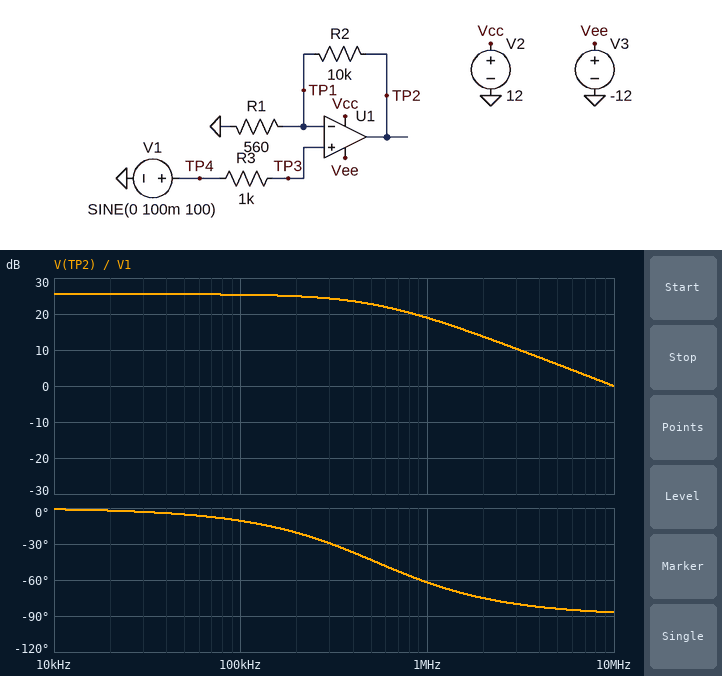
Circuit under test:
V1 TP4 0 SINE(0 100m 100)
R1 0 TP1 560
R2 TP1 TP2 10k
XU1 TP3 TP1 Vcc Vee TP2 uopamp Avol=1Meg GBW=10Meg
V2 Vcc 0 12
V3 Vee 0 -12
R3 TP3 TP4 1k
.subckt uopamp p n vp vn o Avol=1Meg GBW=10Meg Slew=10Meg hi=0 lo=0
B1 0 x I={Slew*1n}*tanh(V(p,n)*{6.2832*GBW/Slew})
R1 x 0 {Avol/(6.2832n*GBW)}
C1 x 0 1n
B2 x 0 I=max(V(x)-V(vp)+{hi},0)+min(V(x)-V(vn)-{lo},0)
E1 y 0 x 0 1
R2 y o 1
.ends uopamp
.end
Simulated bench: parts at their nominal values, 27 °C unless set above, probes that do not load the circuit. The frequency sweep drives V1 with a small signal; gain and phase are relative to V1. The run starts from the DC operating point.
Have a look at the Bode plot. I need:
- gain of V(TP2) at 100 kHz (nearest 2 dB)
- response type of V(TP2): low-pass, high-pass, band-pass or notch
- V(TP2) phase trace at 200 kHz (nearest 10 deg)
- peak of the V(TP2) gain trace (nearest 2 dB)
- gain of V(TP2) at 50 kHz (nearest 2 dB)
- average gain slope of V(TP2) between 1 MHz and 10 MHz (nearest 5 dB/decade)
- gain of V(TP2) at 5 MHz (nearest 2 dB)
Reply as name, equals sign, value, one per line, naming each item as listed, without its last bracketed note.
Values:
gain of V(TP2) at 100 kHz = 26 dB
response type of V(TP2): low-pass, high-pass, band-pass or notch = low-pass
V(TP2) phase trace at 200 kHz = -20 deg
peak of the V(TP2) gain trace = 26 dB
gain of V(TP2) at 50 kHz = 26 dB
average gain slope of V(TP2) between 1 MHz and 10 MHz = -20 dB/decade
gain of V(TP2) at 5 MHz = 6 dB
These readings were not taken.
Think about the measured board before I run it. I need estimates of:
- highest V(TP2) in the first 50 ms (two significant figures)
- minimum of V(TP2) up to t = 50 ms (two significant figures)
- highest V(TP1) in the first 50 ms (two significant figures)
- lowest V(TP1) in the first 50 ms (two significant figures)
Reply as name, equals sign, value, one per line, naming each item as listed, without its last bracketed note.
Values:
highest V(TP2) in the first 50 ms = 1.9 V
minimum of V(TP2) up to t = 50 ms = -1.9 V
highest V(TP1) in the first 50 ms = 100 mV
lowest V(TP1) in the first 50 ms = -100 mV
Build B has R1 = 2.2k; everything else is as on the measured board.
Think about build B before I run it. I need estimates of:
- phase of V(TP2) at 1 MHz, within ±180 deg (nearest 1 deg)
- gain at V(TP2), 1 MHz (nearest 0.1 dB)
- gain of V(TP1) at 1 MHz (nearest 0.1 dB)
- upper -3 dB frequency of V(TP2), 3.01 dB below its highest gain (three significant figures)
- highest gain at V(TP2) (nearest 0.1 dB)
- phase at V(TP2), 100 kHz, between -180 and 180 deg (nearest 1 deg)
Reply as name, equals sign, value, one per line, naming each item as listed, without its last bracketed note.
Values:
phase of V(TP2) at 1 MHz, within ±180 deg = -29 deg
gain at V(TP2), 1 MHz = 13.7 dB
gain of V(TP1) at 1 MHz = -1.2 dB
upper -3 dB frequency of V(TP2), 3.01 dB below its highest gain = 1.80 MHz
highest gain at V(TP2) = 14.9 dB
phase at V(TP2), 100 kHz, between -180 and 180 deg = -3 deg
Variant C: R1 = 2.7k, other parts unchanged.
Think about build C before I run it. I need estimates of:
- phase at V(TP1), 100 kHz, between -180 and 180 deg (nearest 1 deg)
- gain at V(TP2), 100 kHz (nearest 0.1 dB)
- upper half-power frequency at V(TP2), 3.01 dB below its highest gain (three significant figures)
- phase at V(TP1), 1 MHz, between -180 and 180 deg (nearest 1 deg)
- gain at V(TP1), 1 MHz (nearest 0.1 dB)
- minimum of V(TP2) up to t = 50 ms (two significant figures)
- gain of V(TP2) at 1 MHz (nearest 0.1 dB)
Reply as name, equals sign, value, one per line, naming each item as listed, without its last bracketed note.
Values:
phase at V(TP1), 100 kHz, between -180 and 180 deg = -3 deg
gain at V(TP2), 100 kHz = 13.4 dB
upper half-power frequency at V(TP2), 3.01 dB below its highest gain = 2.13 MHz
phase at V(TP1), 1 MHz, between -180 and 180 deg = -25 deg
gain at V(TP1), 1 MHz = -0.9 dB
minimum of V(TP2) up to t = 50 ms = -470 mV
gain of V(TP2) at 1 MHz = 12.6 dB
